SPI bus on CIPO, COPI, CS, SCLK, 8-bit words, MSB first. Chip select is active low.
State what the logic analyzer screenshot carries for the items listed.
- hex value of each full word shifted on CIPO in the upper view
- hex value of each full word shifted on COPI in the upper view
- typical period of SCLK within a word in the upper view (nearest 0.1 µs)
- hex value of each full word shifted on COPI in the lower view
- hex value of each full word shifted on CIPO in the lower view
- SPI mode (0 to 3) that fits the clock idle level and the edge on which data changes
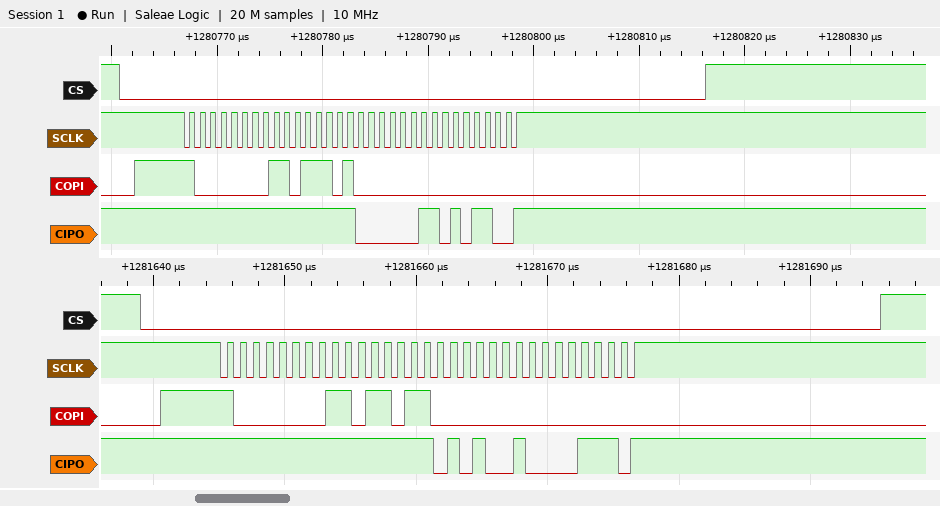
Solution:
FF, FF, 03, 59
80, DD, 00, 00
1 µs
80, DB, 00, 00
FF, FF, 52, 1D
3
